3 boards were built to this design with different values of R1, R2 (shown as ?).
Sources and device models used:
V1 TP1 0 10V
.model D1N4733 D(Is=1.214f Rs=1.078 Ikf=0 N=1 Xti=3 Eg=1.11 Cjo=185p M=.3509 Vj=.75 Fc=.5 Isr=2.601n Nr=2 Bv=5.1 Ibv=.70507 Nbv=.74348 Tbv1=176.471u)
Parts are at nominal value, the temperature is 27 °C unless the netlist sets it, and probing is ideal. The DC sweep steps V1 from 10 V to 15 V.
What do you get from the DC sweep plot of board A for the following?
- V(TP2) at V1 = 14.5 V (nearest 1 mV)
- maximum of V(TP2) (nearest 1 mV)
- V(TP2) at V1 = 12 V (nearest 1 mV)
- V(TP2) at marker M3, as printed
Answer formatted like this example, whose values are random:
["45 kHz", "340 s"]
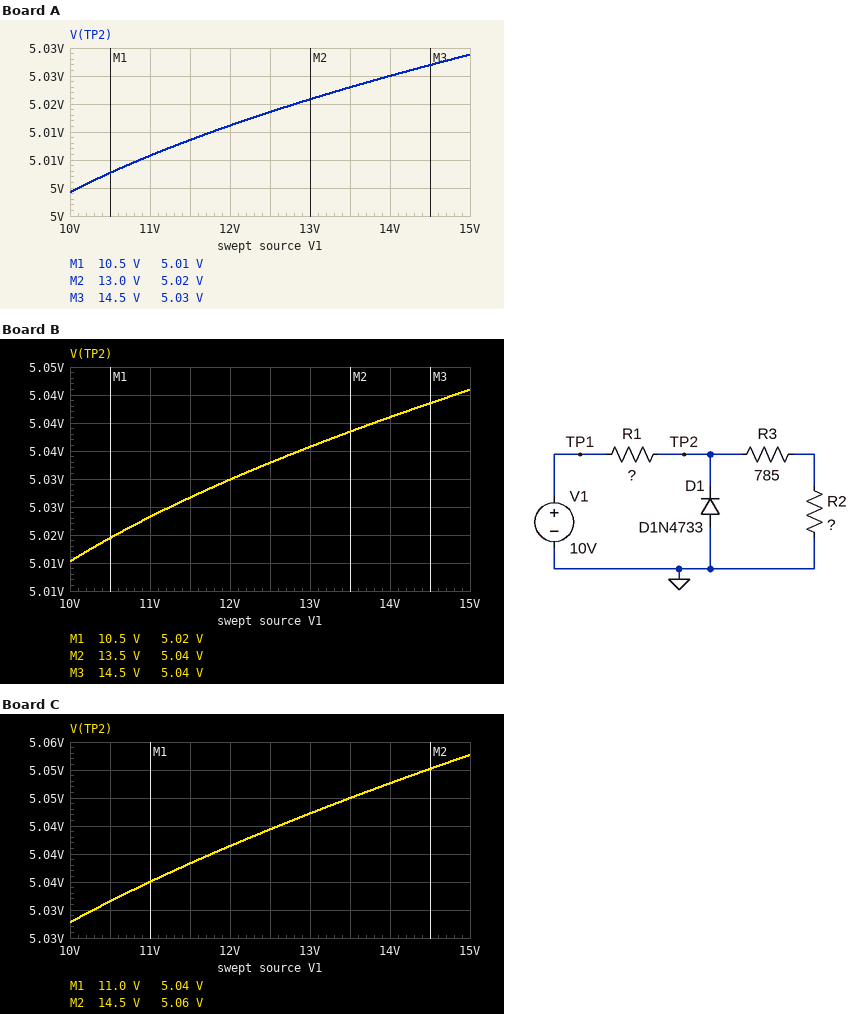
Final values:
["5.027 V", "5.029 V", "5.016 V", "5.03 V"]
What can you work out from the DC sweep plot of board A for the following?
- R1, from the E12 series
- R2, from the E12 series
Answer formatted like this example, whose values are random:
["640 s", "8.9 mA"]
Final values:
["820 Ω", "1.5 kΩ"]
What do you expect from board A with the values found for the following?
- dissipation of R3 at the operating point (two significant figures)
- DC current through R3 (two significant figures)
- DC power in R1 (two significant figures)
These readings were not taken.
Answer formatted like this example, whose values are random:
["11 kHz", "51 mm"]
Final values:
["3.8 mW", "2.2 mA", "30 mW"]
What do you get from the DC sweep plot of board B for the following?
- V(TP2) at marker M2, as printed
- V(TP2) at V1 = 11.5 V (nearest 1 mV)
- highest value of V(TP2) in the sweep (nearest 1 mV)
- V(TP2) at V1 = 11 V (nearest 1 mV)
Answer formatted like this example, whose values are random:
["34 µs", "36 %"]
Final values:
["5.04 V", "5.027 V", "5.046 V", "5.023 V"]
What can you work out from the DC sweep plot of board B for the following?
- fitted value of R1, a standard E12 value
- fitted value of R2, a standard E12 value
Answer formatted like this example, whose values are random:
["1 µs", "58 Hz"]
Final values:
["470 Ω", "330 Ω"]
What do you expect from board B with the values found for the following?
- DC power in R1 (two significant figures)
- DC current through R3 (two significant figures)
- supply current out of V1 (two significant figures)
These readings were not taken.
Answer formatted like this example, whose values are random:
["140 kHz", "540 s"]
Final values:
["53 mW", "4.5 mA", "11 mA"]
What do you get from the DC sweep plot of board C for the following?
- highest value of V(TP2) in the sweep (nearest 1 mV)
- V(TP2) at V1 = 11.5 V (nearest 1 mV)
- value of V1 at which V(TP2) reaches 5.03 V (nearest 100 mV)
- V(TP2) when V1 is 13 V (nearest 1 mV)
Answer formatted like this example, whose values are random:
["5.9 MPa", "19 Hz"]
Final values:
["5.058 V", "5.038 V", "10.3 V", "5.047 V"]
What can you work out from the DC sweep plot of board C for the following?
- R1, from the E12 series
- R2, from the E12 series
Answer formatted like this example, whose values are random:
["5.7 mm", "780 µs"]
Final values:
["390 Ω", "820 Ω"]
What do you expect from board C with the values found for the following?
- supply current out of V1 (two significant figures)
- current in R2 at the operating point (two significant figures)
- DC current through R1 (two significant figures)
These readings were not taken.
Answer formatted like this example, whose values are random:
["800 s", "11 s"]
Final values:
["13 mA", "3.1 mA", "13 mA"]
